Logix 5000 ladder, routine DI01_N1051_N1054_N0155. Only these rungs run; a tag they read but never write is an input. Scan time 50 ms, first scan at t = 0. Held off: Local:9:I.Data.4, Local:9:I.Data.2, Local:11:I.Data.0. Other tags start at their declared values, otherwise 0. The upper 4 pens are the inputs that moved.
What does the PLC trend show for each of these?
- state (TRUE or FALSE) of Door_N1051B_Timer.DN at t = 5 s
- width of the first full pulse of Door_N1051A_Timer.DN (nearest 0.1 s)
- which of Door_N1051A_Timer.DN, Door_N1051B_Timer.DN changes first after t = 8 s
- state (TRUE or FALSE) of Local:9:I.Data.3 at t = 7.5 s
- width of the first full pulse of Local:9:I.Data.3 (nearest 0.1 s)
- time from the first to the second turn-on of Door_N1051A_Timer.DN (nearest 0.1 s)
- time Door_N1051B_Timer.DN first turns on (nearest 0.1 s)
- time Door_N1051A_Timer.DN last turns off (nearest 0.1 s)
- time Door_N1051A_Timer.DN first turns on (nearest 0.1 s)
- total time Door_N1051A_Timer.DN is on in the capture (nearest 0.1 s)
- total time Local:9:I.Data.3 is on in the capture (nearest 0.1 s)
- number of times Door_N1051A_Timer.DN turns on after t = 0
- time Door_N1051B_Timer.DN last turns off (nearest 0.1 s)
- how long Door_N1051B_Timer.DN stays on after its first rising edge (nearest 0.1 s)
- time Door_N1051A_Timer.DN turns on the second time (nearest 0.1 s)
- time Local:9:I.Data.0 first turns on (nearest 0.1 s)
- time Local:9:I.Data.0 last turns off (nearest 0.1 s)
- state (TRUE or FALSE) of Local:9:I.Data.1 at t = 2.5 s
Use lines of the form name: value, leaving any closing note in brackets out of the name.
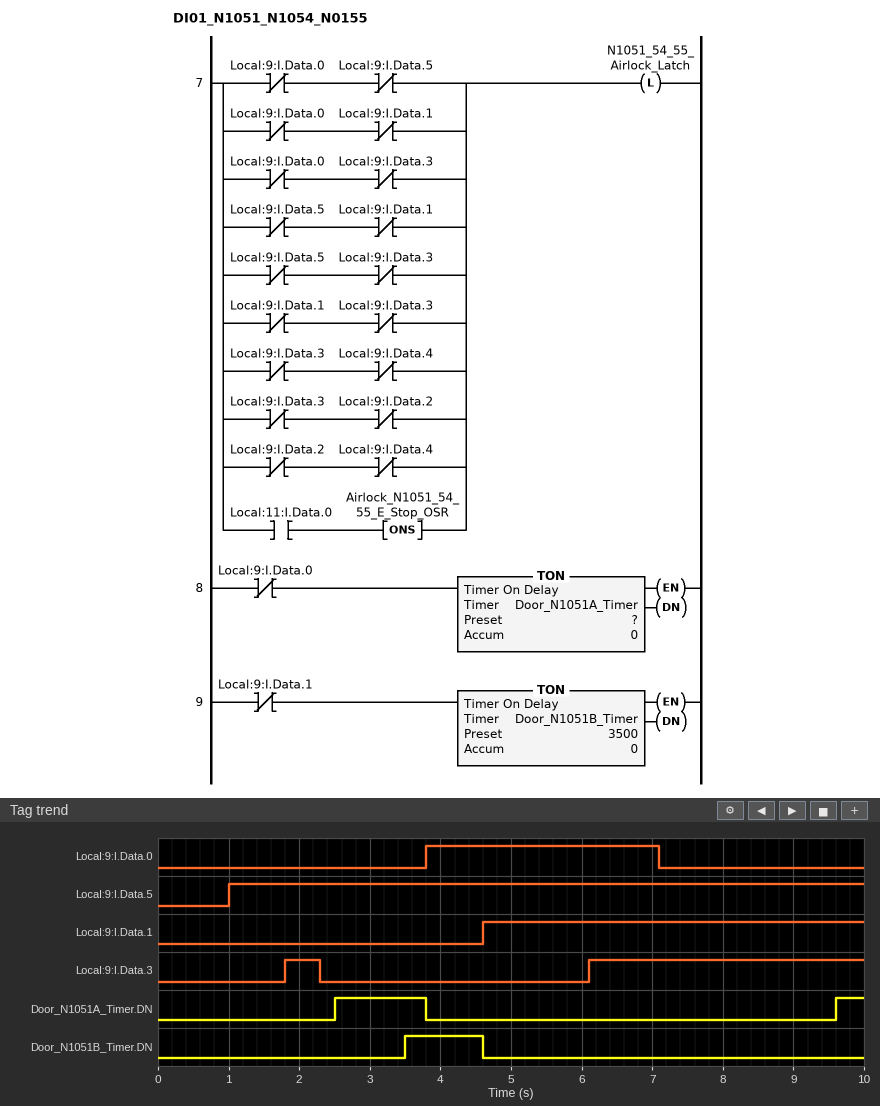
state (TRUE or FALSE) of Door_N1051B_Timer.DN at t = 5 s: FALSE
width of the first full pulse of Door_N1051A_Timer.DN: 1.3 s
which of Door_N1051A_Timer.DN, Door_N1051B_Timer.DN changes first after t = 8 s: Door_N1051A_Timer.DN
state (TRUE or FALSE) of Local:9:I.Data.3 at t = 7.5 s: TRUE
width of the first full pulse of Local:9:I.Data.3: 0.5 s
time from the first to the second turn-on of Door_N1051A_Timer.DN: 7.1 s
time Door_N1051B_Timer.DN first turns on: 3.5 s
time Door_N1051A_Timer.DN last turns off: 3.8 s
time Door_N1051A_Timer.DN first turns on: 2.5 s
total time Door_N1051A_Timer.DN is on in the capture: 1.7 s
total time Local:9:I.Data.3 is on in the capture: 4.4 s
number of times Door_N1051A_Timer.DN turns on after t = 0: 2
time Door_N1051B_Timer.DN last turns off: 4.6 s
how long Door_N1051B_Timer.DN stays on after its first rising edge: 1.1 s
time Door_N1051A_Timer.DN turns on the second time: 9.6 s
time Local:9:I.Data.0 first turns on: 3.8 s
time Local:9:I.Data.0 last turns off: 7.1 s
state (TRUE or FALSE) of Local:9:I.Data.1 at t = 2.5 s: FALSE
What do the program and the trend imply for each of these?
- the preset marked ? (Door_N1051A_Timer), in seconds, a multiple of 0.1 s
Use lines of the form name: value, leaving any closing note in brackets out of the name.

the preset marked ? (Door_N1051A_Timer), in seconds, a multiple of 0.1 s: 2.5 s
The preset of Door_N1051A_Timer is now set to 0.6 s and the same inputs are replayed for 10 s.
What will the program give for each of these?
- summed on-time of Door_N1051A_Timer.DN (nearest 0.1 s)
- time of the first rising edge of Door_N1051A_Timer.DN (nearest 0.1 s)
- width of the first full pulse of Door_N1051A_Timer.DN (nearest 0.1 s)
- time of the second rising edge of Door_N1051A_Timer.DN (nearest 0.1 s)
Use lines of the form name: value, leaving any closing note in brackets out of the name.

summed on-time of Door_N1051A_Timer.DN: 5.5 s
time of the first rising edge of Door_N1051A_Timer.DN: 0.6 s
width of the first full pulse of Door_N1051A_Timer.DN: 3.2 s
time of the second rising edge of Door_N1051A_Timer.DN: 7.7 s
